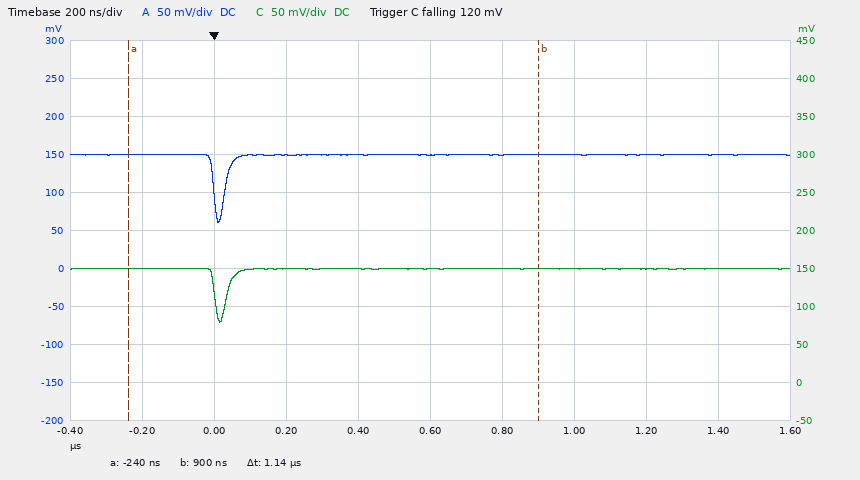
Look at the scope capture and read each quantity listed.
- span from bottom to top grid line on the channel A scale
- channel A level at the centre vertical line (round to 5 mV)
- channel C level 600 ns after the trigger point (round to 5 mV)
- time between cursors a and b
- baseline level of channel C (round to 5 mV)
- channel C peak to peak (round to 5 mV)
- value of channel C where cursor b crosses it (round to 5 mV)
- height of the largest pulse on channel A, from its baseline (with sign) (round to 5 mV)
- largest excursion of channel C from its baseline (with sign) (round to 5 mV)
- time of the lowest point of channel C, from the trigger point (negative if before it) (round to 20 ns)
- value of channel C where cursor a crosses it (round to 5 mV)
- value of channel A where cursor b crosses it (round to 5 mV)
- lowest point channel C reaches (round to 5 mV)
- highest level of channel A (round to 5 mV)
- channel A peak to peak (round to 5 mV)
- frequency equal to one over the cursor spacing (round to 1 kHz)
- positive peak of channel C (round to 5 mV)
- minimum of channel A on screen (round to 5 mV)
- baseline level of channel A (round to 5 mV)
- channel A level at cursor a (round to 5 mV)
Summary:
500 mV
150 mV
150 mV
1.14 µs
150 mV
70 mV
150 mV
-90 mV
-70 mV
+20 ns
150 mV
150 mV
80 mV
150 mV
90 mV
877 kHz
150 mV
60 mV
150 mV
150 mV
